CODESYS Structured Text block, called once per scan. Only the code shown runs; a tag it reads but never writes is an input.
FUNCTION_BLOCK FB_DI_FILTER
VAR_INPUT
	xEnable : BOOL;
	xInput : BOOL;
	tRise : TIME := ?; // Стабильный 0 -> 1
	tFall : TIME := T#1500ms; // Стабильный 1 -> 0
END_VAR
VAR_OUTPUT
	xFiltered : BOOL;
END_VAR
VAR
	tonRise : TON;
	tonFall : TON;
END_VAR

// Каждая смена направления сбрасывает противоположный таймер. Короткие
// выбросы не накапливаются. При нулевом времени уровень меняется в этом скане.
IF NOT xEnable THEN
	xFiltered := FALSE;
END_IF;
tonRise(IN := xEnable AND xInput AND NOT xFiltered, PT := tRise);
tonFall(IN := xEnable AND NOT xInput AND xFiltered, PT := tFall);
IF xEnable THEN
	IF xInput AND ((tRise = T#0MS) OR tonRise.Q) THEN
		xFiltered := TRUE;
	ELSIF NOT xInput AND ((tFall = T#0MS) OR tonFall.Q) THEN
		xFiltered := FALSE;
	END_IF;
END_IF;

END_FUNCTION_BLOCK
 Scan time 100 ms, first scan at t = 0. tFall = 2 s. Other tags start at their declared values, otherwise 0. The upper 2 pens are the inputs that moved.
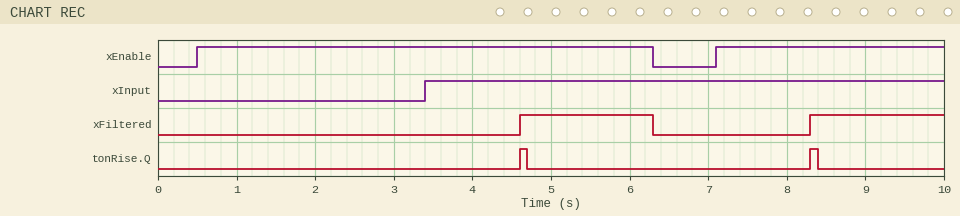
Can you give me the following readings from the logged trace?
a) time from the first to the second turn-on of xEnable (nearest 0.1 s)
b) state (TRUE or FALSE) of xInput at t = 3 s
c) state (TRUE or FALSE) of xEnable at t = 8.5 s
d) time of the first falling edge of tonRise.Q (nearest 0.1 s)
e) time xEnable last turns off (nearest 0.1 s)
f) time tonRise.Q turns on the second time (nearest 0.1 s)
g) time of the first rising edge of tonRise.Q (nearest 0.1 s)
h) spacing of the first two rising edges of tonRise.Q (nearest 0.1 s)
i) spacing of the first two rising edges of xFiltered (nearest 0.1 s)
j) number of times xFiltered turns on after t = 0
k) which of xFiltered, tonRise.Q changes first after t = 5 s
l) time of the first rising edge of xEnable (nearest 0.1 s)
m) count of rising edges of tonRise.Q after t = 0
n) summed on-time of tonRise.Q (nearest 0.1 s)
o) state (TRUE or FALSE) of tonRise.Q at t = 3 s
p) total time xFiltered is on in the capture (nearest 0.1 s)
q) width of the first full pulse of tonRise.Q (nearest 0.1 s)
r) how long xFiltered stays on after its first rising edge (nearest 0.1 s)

6.6 s
FALSE
TRUE
4.7 s
6.3 s
8.3 s
4.6 s
3.7 s
3.7 s
2
xFiltered
0.5 s
2
0.2 s
FALSE
3.4 s
0.1 s
1.7 s
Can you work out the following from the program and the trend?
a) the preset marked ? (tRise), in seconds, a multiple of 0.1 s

1.2 s
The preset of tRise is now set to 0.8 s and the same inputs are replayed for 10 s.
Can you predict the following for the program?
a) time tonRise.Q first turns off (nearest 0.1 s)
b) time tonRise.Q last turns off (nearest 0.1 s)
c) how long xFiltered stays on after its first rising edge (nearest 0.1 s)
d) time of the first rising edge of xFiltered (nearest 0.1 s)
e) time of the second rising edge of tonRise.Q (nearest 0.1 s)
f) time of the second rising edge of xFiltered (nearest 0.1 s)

4.3 s
8.0 s
2.1 s
4.2 s
7.9 s
7.9 s
